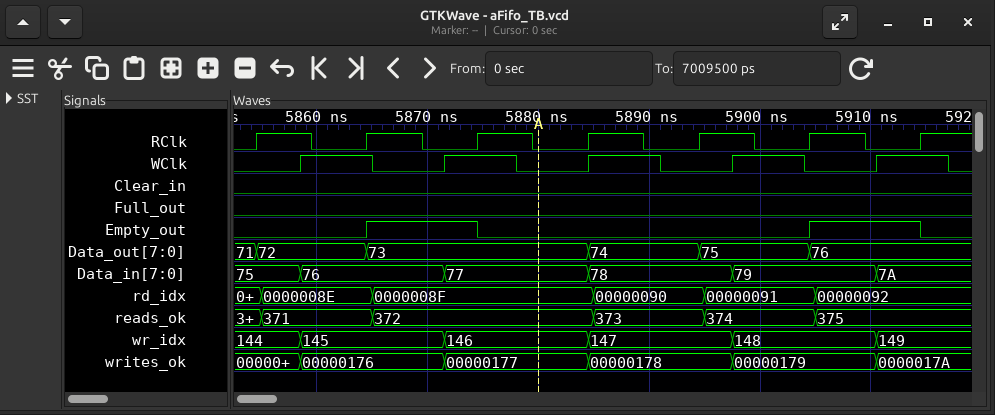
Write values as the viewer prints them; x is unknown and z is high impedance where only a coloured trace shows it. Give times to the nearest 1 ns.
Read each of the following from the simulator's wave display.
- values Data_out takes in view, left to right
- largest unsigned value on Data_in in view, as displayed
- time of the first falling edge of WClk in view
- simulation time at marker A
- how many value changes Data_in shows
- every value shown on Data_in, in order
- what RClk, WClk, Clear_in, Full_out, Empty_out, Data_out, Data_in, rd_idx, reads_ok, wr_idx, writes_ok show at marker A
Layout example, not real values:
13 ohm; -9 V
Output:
71, 72, 73, 74, 75, 76; 7A; 5865 ns; 5880 ns; 5; 75, 76, 77, 78, 79, 7A; RClk=0, WClk=0, Clear_in=0, Full_out=0, Empty_out=0, Data_out=73, Data_in=77, rd_idx=0000008F, reads_ok=372, wr_idx=146, writes_ok=00000177
